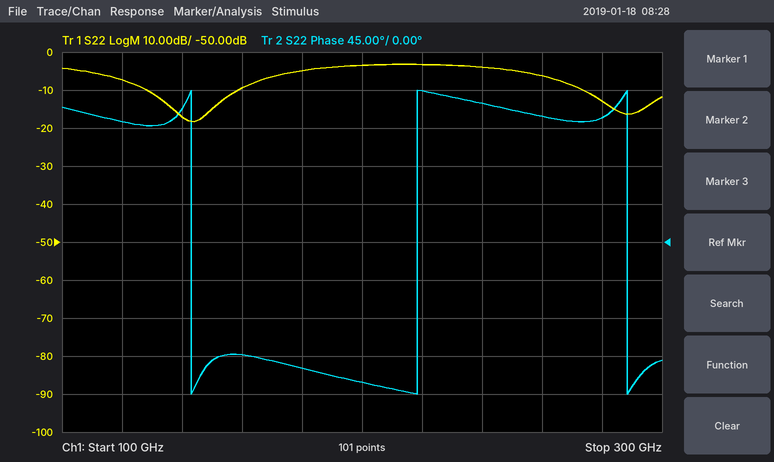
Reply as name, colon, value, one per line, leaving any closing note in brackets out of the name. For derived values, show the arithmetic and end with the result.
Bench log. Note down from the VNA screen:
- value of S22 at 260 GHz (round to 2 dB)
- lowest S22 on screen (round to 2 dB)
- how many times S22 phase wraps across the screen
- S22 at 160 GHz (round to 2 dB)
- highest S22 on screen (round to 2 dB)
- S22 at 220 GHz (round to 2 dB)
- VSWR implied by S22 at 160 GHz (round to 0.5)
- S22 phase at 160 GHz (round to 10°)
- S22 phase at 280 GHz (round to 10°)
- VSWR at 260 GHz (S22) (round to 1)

value of S22 at 260 GHz: -6 dB
lowest S22 on screen: -18 dB
how many times S22 phase wraps across the screen: 3
S22 at 160 GHz: -10 dB
highest S22 on screen: -4 dB
S22 at 220 GHz: -4 dB
VSWR implied by S22 at 160 GHz: |Γ| = 10^(-10/20) = 0.3162; VSWR = (1 + 0.3162)/(1 − 0.3162) ≈ 1.92, so 2.0 to the nearest 0.5
S22 phase at 160 GHz: -130°
S22 phase at 280 GHz: 150°
VSWR at 260 GHz (S22): |Γ| = 10^(-6/20) = 0.5012; VSWR = (1 + 0.5012)/(1 − 0.5012) ≈ 3
